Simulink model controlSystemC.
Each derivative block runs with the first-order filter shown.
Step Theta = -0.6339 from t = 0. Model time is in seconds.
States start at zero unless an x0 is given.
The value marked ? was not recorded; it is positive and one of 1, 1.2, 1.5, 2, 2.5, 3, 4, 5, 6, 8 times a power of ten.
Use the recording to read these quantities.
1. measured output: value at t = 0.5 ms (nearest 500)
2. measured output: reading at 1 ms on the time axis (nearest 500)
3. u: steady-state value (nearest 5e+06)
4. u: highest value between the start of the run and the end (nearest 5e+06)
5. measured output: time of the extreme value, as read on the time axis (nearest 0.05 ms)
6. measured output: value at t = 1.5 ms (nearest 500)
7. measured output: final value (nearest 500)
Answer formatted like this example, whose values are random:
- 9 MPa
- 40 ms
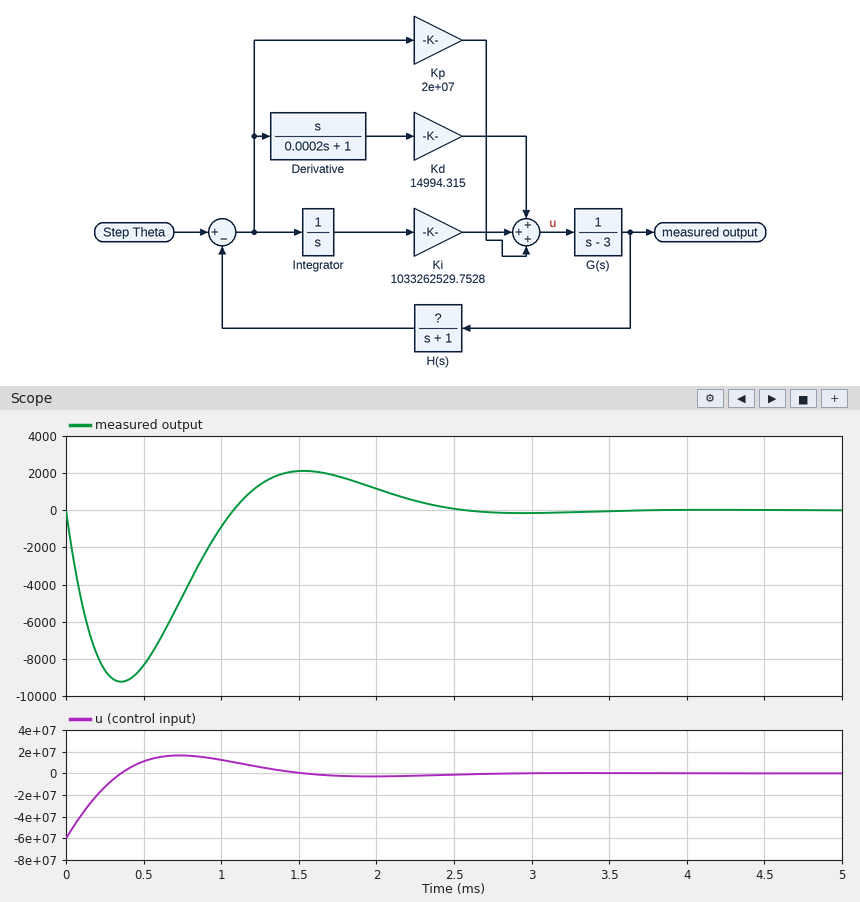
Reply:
- -8500
- -1000
- 0
- 15000000
- 0.35 ms
- 2000
- 0
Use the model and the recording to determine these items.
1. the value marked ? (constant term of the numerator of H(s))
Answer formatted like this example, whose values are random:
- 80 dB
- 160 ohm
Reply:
- 0.15
